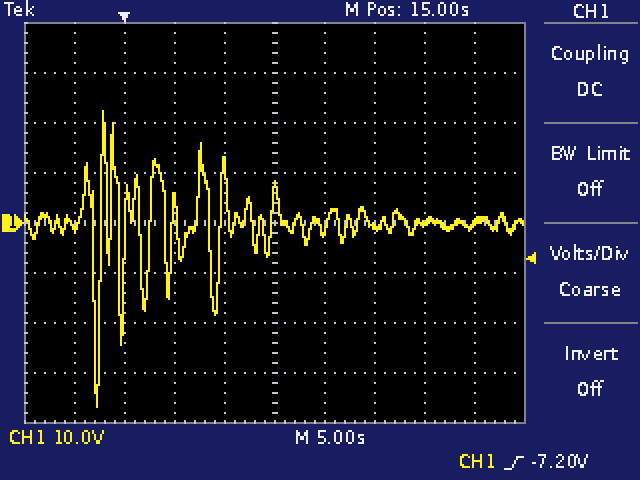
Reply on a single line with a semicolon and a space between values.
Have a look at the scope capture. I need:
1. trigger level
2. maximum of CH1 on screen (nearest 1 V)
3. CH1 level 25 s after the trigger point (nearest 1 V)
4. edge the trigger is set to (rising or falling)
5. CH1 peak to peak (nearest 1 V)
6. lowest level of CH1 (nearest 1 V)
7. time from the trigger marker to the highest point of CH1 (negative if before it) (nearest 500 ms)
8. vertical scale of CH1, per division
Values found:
-7.20 V; 22 V; -1 V; rising; 59 V; -37 V; -2.0 s; 10 V
